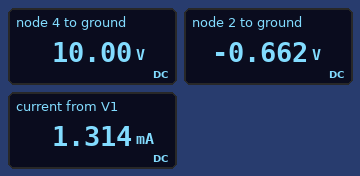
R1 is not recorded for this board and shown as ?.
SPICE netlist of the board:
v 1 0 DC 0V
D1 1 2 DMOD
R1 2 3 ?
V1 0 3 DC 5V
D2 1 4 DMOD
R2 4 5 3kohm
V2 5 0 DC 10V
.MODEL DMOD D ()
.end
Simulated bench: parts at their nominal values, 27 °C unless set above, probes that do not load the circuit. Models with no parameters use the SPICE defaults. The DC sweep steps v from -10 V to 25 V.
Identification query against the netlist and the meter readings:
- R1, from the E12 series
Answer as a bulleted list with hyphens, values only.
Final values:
- 3.3 kΩ
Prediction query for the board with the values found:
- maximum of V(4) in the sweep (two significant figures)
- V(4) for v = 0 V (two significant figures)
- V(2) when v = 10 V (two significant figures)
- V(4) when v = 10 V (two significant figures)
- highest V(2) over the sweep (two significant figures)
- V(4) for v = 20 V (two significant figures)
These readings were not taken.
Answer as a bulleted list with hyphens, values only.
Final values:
- 24 V
- 10 V
- 9.3 V
- 10 V
- 24 V
- 19 V
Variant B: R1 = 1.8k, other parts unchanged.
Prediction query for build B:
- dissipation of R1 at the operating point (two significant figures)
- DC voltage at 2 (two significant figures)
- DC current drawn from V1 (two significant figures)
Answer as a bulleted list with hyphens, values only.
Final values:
- 10 mW
- -680 mV
- 2.4 mA
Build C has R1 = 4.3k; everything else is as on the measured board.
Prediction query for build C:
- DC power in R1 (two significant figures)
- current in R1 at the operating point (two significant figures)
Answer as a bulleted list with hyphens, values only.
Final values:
- 4.4 mW
- 1.0 mA
